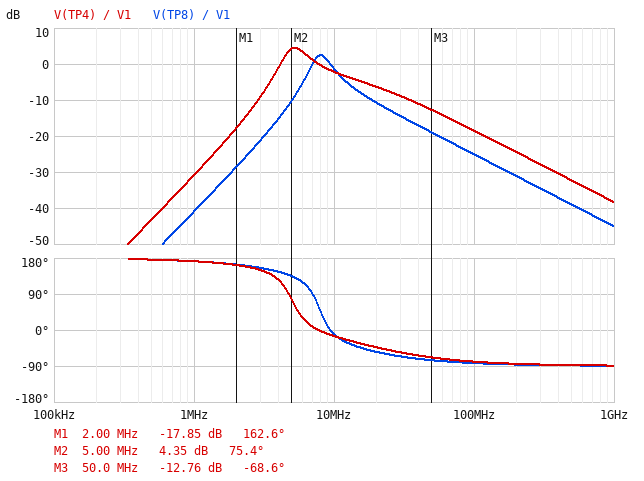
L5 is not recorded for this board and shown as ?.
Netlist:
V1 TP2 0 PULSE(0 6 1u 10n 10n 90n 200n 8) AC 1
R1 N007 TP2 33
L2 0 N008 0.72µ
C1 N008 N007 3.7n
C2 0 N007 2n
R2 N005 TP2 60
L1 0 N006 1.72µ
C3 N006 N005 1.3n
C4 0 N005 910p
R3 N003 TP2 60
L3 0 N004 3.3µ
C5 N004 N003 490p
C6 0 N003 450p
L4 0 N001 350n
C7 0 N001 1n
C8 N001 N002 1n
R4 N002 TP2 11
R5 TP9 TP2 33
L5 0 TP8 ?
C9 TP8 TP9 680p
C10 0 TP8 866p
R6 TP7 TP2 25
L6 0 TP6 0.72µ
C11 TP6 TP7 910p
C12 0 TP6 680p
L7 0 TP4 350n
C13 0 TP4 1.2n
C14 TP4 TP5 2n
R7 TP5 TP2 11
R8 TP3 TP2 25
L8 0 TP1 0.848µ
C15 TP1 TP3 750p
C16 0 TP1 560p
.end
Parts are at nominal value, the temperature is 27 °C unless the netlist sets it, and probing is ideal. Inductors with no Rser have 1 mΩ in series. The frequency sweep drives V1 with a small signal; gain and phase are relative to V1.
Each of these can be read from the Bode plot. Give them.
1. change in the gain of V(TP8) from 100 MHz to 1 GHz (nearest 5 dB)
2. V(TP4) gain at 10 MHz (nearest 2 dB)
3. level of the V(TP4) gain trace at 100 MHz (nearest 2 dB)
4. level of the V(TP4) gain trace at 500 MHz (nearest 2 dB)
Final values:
-20 dB
-2 dB
-18 dB
-32 dB
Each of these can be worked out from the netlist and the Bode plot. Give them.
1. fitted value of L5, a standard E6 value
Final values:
330 nH
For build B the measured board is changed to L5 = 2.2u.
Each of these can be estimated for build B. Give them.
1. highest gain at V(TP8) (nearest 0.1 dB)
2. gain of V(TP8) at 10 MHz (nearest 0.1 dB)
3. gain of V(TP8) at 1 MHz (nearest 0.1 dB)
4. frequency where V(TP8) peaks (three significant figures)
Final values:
8.7 dB
-8.4 dB
-23.4 dB
2.80 MHz
